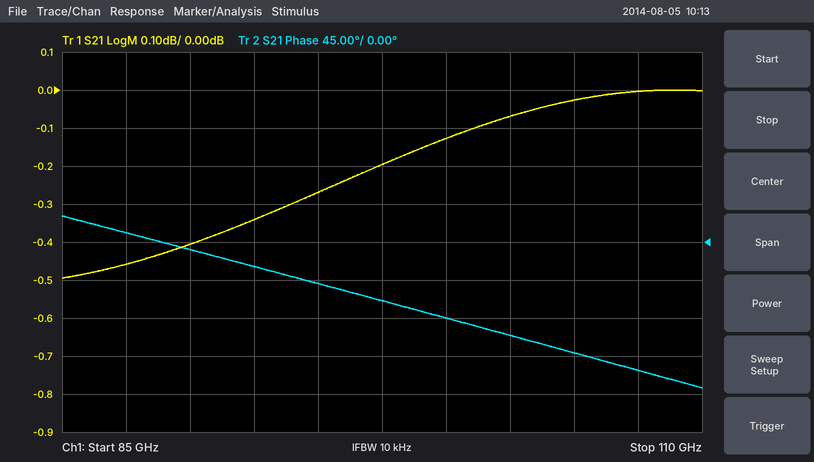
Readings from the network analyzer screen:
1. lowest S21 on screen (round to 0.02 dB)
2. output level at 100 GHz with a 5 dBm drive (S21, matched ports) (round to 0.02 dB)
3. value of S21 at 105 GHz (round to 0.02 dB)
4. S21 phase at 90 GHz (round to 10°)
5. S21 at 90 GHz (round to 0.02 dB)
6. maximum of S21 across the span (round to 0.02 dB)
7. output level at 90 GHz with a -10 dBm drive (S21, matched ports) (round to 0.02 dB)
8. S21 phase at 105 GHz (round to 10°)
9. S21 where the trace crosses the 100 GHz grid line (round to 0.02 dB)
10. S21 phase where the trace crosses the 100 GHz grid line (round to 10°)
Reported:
-0.50 dB
4.88 dBm
-0.02 dB
-10°
-0.40 dB
0.00 dB
-10.40 dBm
-130°
-0.12 dB
-90°
